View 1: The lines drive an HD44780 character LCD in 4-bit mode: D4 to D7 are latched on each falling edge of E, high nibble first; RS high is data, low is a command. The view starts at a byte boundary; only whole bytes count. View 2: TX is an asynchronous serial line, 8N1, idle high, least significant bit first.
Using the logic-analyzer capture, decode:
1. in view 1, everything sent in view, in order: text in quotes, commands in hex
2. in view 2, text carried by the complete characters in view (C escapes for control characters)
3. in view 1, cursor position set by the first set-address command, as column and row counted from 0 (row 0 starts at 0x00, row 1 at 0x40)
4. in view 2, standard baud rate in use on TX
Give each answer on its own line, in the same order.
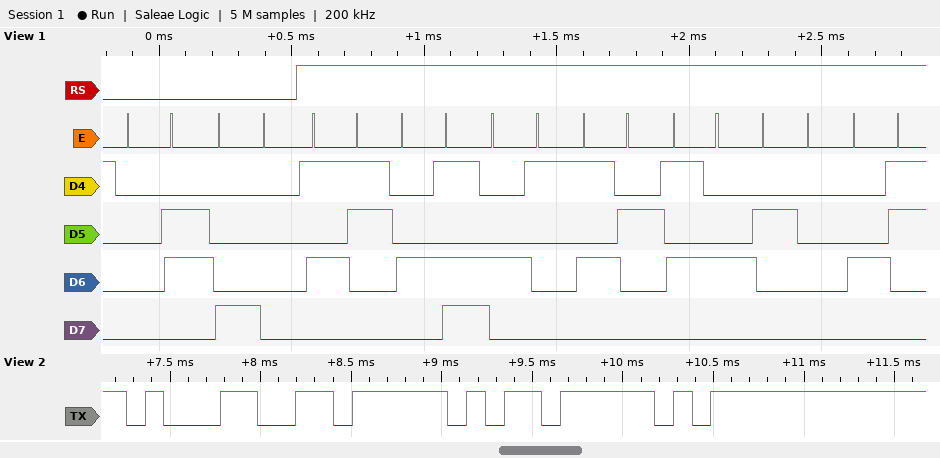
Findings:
0x06 0x80 "SMART C"
"1__"
column 0, row 0
9600 baud
